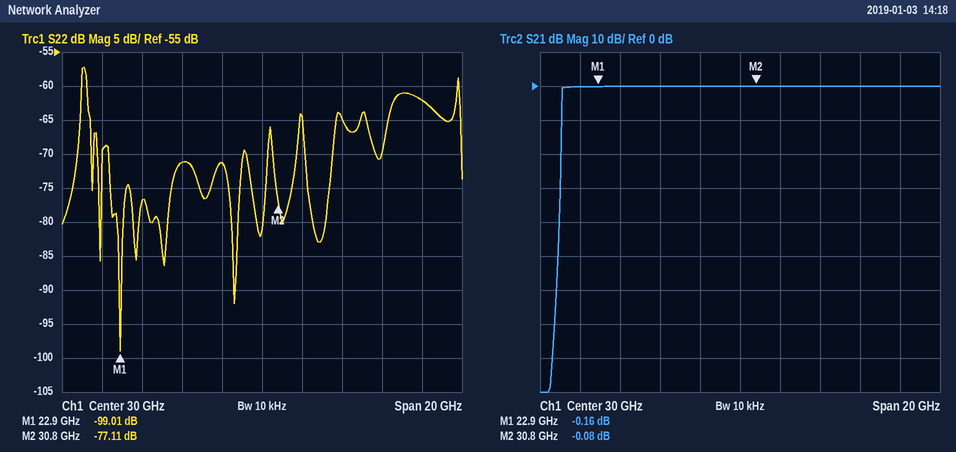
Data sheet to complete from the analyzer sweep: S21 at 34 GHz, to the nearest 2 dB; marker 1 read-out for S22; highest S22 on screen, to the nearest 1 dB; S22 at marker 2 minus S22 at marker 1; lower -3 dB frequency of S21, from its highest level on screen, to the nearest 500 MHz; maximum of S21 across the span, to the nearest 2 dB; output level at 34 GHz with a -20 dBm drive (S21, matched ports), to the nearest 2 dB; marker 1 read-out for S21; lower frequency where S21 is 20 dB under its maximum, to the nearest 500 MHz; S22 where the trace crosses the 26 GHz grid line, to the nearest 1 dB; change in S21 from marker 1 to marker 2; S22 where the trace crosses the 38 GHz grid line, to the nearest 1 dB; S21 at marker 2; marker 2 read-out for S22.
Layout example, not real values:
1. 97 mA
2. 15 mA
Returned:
1. 0 dB
2. -99.01 dB
3. -57 dB
4. 21.90 dB
5. 21.0 GHz
6. 0 dB
7. -20 dBm
8. -0.16 dB
9. 21.0 GHz
10. -71 dB
11. 0.08 dB
12. -62 dB
13. -0.08 dB
14. -77.11 dB
